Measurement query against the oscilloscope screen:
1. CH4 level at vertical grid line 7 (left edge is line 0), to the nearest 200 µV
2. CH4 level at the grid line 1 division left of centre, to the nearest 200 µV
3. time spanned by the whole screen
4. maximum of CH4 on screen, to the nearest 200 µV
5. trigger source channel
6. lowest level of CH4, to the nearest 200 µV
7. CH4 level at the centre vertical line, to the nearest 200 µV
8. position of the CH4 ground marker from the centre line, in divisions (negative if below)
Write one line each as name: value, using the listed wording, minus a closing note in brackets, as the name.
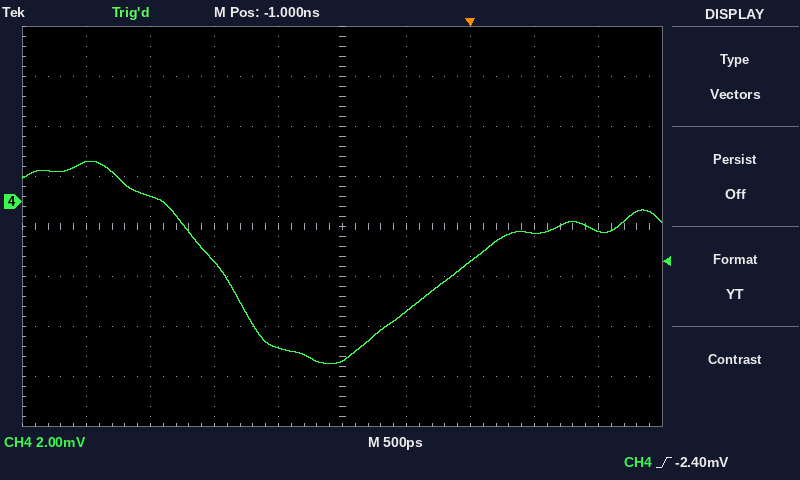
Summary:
CH4 level at vertical grid line 7 (left edge is line 0), to the nearest 200 µV: -2.4 mV
CH4 level at the grid line 1 division left of centre, to the nearest 200 µV: -5.8 mV
time spanned by the whole screen: 5 ns
maximum of CH4 on screen, to the nearest 200 µV: 1.6 mV
trigger source channel: CH4
lowest level of CH4, to the nearest 200 µV: -6.4 mV
CH4 level at the centre vertical line, to the nearest 200 µV: -6.4 mV
position of the CH4 ground marker from the centre line, in divisions: +0.5 div
